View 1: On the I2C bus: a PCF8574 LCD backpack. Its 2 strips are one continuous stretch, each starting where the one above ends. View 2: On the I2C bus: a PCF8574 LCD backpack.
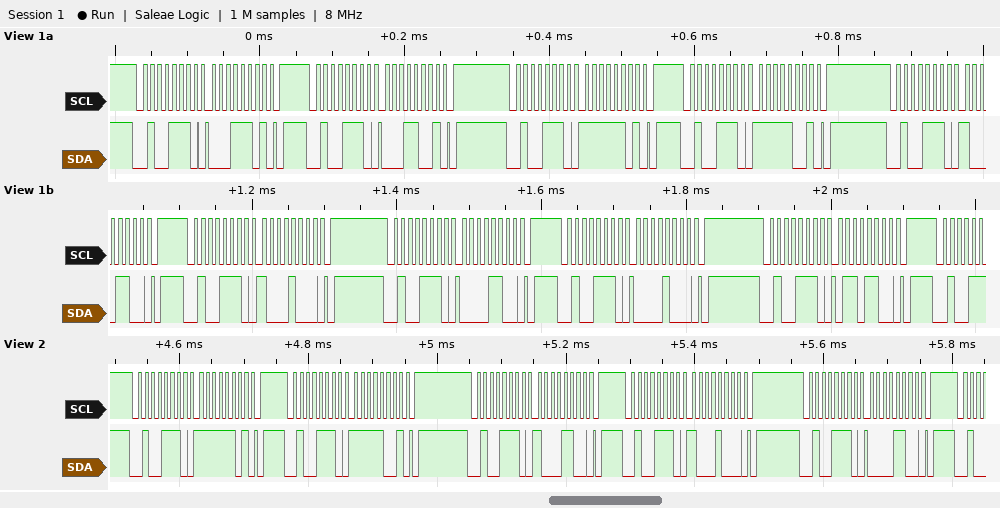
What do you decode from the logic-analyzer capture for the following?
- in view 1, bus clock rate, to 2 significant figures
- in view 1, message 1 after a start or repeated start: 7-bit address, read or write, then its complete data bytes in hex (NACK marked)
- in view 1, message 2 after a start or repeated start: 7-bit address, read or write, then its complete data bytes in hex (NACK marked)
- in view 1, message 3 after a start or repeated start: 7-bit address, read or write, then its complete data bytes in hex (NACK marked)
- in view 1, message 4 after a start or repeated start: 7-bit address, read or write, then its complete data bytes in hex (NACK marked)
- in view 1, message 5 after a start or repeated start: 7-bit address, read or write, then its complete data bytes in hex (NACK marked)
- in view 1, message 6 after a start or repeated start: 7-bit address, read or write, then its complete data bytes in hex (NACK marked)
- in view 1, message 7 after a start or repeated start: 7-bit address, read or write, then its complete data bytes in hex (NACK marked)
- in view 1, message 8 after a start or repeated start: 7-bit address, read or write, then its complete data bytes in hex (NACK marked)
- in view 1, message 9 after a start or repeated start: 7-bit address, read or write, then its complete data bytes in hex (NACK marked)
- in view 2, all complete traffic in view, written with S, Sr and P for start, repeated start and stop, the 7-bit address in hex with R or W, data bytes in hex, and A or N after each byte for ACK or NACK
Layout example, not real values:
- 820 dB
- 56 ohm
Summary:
- 100 kHz
- 0x27 write: 1D
- 0x27 write: 19
- 0x27 write: FD
- 0x27 write: F9
- 0x27 write: 8C
- 0x27 write: 88
- 0x27 write: 0C
- 0x27 write: 08
- 0x27 write: 6C
- S 27W A FD A P S 27W A F9 A P S 27W A 8C A P S 27W A 88 A P S 27W A 0C A P
